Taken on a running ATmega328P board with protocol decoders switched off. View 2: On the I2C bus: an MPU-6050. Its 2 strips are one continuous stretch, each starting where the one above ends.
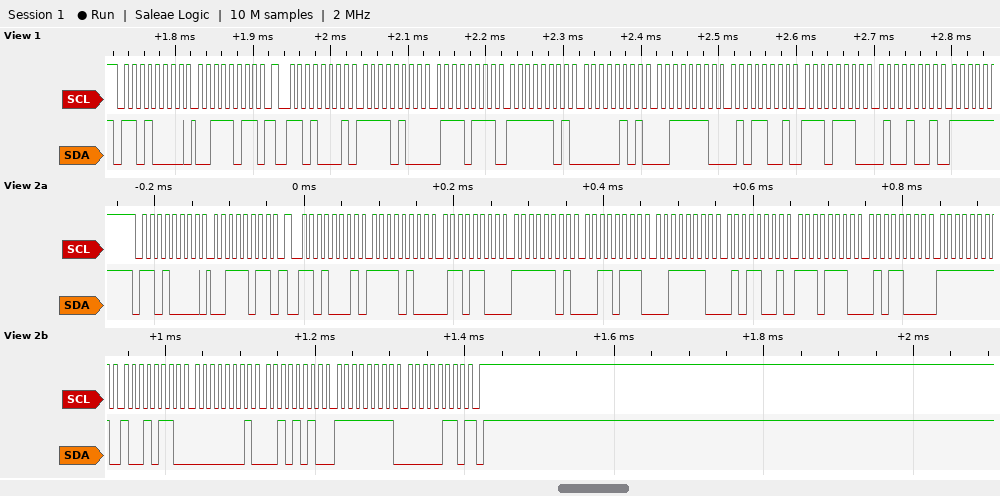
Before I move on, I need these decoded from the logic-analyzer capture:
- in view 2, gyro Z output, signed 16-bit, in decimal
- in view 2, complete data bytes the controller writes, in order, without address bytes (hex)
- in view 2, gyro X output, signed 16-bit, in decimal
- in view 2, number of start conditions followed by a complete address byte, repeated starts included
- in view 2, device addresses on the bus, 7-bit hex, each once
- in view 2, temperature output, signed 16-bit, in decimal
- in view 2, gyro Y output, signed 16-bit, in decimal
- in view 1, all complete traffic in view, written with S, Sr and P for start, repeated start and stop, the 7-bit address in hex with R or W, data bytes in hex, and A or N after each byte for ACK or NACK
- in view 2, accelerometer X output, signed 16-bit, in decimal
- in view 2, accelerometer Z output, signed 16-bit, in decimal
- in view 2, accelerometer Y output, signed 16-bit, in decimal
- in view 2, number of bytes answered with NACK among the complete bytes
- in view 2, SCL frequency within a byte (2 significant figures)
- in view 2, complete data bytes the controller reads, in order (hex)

-250
3B
-106
2
0x68
-4520
298
S 68W A 3B A Sr 68R A F4 A 77 A FD A 05 A 3E A 59 A EE A 49 A
-2964
15961
-713
1
100 kHz
F4 6C FD 37 3E 59 EE 58 FF 96 01 2A FF 06
